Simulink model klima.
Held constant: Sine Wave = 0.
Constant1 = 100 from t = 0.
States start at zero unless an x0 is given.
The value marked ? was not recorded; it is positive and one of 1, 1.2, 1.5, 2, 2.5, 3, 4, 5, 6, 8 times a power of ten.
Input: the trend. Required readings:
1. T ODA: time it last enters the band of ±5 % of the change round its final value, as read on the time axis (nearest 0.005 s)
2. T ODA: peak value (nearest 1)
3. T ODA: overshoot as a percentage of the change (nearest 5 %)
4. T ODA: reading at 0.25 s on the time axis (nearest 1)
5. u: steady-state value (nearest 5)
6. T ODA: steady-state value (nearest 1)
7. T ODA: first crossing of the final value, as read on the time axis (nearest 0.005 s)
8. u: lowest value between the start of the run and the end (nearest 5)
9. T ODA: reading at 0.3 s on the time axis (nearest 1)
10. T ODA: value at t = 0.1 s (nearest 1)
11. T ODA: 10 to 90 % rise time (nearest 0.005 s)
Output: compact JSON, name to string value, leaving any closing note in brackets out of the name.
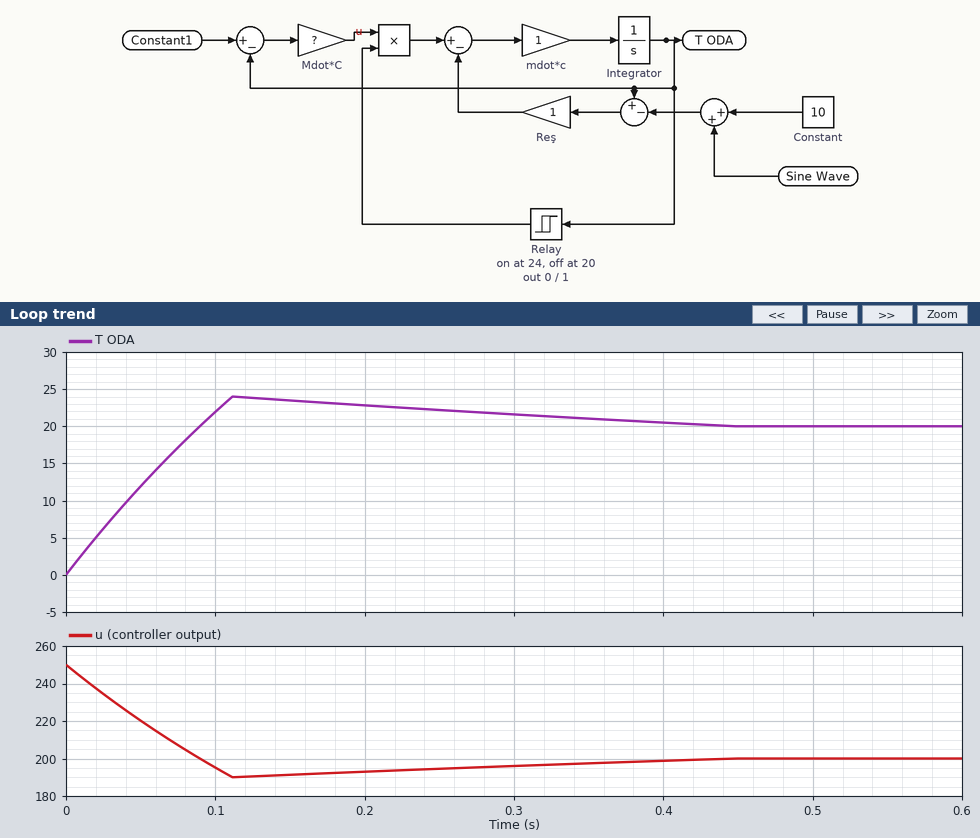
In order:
{"T ODA: time it last enters the band of ±5 % of the change round its final value, as read on the time axis": "0.350 s", "T ODA: peak value": "24", "T ODA: overshoot as a percentage of the change": "20 %", "T ODA: reading at 0.25 s on the time axis": "22", "u: steady-state value": "200", "T ODA: steady-state value": "20", "T ODA: first crossing of the final value, as read on the time axis": "0.090 s", "u: lowest value between the start of the run and the end": "190", "T ODA: reading at 0.3 s on the time axis": "22", "T ODA: value at t = 0.1 s": "22", "T ODA: 10 to 90 % rise time": "0.070 s"}
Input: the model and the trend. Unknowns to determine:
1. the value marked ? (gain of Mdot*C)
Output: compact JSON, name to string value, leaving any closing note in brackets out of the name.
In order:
{"the value marked ?": "2.5"}
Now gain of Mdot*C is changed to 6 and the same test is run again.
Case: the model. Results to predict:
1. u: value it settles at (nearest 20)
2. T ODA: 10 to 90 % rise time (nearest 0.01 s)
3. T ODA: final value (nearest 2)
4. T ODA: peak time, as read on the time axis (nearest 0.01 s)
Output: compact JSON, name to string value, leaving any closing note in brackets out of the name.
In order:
{"u: value it settles at": "480", "T ODA: 10 to 90 % rise time": "0.03 s", "T ODA: final value": "20", "T ODA: peak time, as read on the time axis": "0.05 s"}
